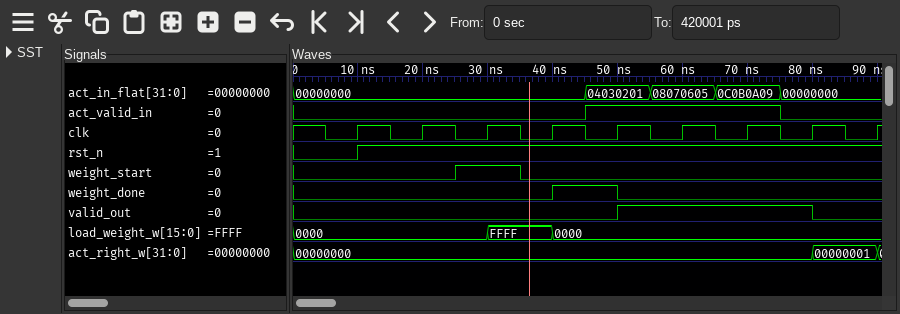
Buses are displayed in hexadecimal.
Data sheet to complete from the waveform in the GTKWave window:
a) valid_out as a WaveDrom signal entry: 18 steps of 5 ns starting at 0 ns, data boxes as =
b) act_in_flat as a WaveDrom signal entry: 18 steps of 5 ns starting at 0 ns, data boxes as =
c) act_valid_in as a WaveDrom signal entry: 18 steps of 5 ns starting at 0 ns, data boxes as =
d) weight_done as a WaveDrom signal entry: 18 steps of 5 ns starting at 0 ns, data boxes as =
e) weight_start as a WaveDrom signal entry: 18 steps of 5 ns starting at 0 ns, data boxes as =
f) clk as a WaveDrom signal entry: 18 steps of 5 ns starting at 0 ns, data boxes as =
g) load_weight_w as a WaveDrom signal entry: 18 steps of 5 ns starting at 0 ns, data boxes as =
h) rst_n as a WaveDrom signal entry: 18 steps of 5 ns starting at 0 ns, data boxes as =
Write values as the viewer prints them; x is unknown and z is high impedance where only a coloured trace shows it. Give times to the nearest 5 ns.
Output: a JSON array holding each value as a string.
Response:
["{name: 'valid_out', wave: '0.........1.....0.'}", "{name: 'act_in_flat', wave: '=........=.=.=.=..', data: '00000000 04030201 08070605 0C0B0A09 00000000'}", "{name: 'act_valid_in', wave: '0........1.....0..'}", "{name: 'weight_done', wave: '0.......1.0.......'}", "{name: 'weight_start', wave: '0....1.0..........'}", "{name: 'clk', wave: '101010101010101010'}", "{name: 'load_weight_w', wave: '=.....=.=.........', data: '0000 FFFF 0000'}", "{name: 'rst_n', wave: '0.1...............'}"]
